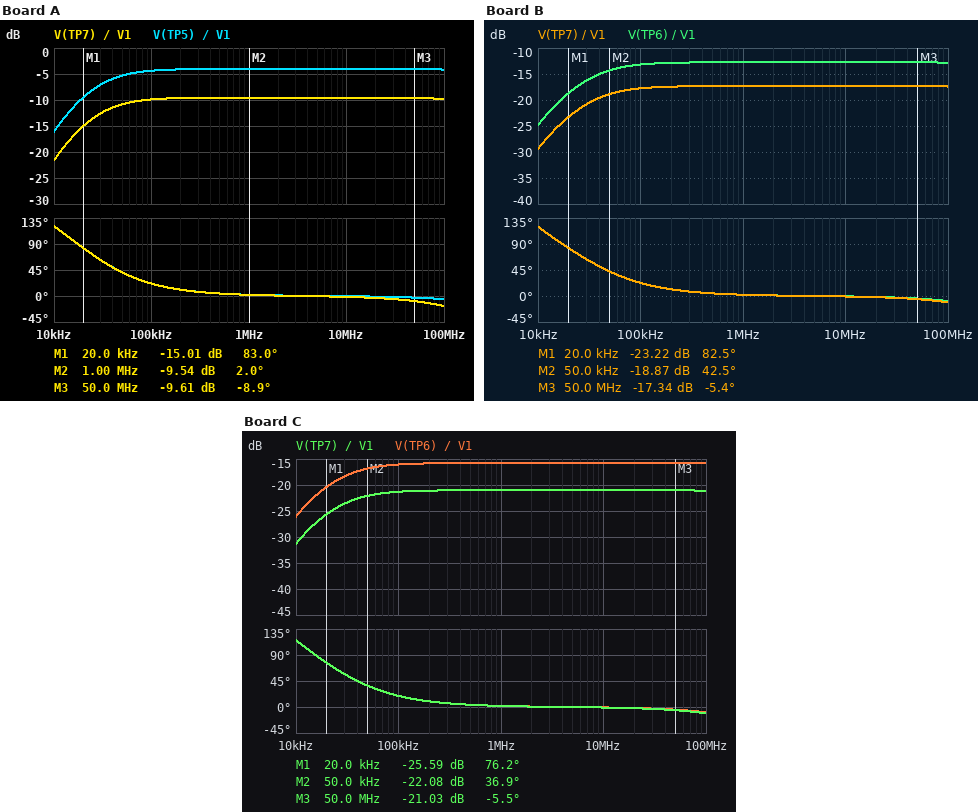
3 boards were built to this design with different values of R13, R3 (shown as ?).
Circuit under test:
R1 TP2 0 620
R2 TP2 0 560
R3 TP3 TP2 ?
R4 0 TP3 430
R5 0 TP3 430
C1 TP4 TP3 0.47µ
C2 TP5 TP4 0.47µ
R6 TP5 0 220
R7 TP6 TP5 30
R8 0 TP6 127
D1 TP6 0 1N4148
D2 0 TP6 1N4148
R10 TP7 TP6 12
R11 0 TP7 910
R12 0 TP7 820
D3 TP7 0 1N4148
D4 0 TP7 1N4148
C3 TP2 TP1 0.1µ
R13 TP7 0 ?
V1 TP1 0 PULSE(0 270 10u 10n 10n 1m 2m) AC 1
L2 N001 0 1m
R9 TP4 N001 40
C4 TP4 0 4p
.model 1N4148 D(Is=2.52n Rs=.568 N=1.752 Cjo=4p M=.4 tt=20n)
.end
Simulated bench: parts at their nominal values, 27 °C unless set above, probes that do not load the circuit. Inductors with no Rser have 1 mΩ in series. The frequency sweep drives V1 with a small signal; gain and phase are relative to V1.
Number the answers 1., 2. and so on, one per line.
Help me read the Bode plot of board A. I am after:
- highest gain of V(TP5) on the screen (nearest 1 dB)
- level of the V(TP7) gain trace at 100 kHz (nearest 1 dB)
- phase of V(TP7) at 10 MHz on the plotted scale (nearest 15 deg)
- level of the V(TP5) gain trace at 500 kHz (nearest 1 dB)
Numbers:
1. -4 dB
2. -10 dB
3. 0 deg
4. -4 dB
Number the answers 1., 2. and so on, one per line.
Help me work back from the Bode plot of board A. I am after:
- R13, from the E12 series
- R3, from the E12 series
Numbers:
1. 82 Ω
2. 27 Ω
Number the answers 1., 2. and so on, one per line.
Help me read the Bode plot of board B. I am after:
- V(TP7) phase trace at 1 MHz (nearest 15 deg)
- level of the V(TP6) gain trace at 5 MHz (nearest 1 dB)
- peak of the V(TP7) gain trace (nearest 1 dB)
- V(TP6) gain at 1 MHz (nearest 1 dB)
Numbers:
1. 0 deg
2. -13 dB
3. -17 dB
4. -13 dB
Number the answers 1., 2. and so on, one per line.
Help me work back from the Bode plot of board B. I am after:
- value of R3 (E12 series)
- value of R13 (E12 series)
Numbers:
1. 33 Ω
2. 18 Ω
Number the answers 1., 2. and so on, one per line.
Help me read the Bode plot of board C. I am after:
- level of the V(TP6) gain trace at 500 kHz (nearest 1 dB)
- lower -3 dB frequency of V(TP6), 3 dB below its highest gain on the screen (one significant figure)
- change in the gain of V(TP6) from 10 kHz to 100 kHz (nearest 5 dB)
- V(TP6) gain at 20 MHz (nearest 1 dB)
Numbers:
1. -16 dB
2. 30 kHz
3. 10 dB
4. -16 dB
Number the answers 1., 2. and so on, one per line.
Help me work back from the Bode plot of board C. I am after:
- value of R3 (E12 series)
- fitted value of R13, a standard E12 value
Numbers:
1. 56 Ω
2. 15 Ω
